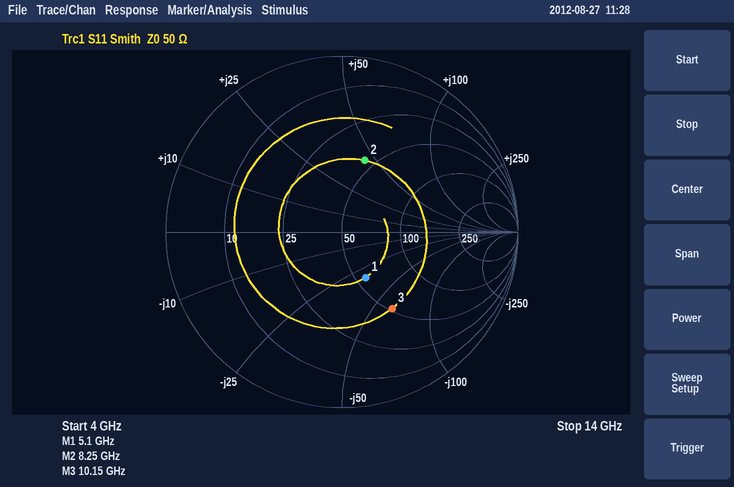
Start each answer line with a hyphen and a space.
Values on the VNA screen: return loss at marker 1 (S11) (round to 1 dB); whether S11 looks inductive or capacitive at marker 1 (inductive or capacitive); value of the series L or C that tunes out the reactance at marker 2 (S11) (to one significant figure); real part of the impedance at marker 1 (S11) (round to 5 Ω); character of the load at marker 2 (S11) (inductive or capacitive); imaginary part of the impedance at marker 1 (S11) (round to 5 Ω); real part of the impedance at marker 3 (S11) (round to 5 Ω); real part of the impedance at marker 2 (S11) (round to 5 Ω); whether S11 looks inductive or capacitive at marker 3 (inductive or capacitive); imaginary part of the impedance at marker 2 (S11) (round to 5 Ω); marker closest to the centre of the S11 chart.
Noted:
- 11 dB
- capacitive
- 400 fF
- 55 Ω
- inductive
- -30 Ω
- 50 Ω
- 45 Ω
- capacitive
- +45 Ω
- marker 1
